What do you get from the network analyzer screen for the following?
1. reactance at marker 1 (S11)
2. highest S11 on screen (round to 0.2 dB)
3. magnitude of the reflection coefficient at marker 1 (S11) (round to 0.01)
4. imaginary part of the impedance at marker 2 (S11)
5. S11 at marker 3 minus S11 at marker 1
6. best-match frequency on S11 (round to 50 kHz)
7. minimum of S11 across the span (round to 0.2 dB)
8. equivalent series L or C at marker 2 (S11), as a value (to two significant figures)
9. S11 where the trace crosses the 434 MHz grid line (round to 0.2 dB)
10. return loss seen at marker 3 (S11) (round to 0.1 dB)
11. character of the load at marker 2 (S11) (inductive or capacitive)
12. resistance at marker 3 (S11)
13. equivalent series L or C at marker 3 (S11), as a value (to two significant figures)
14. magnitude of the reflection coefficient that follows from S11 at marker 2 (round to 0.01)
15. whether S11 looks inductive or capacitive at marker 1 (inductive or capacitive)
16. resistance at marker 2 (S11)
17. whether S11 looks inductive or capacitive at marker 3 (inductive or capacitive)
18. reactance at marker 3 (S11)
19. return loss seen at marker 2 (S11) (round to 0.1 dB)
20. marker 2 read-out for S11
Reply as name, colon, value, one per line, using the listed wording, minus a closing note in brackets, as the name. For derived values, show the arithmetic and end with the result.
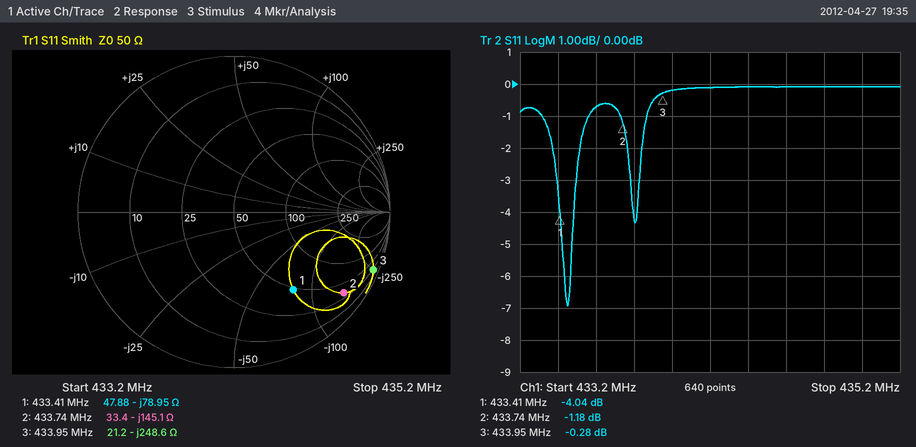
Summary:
reactance at marker 1: -78.95 Ω
highest S11 on screen: 0.0 dB
magnitude of the reflection coefficient at marker 1 (S11): 0.63
imaginary part of the impedance at marker 2: -145.1 Ω
S11 at marker 3 minus S11 at marker 1: -0.28 − (-4.04) = 3.76 dB
best-match frequency on S11: 433.45 MHz
minimum of S11 across the span: -7.0 dB
equivalent series L or C at marker 2 (S11), as a value: C = 1/(2π × 433.74 MHz × 145.1 Ω) ≈ 2.5 pF
S11 where the trace crosses the 434 MHz grid line: -0.2 dB
return loss seen at marker 3 (S11): 0.3 dB
character of the load at marker 2 (S11): capacitive
resistance at marker 3: 21.2 Ω
equivalent series L or C at marker 3 (S11), as a value: C = 1/(2π × 433.95 MHz × 248.6 Ω) ≈ 1.5 pF
magnitude of the reflection coefficient that follows from S11 at marker 2: 10^(-1.18/20) ≈ 0.87
whether S11 looks inductive or capacitive at marker 1: capacitive
resistance at marker 2: 33.4 Ω
whether S11 looks inductive or capacitive at marker 3: capacitive
reactance at marker 3: -248.6 Ω
return loss seen at marker 2 (S11): 1.2 dB
marker 2 read-out for S11: -1.18 dB
